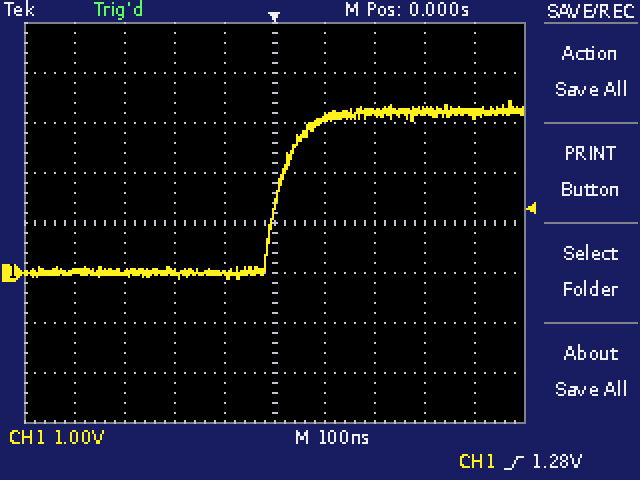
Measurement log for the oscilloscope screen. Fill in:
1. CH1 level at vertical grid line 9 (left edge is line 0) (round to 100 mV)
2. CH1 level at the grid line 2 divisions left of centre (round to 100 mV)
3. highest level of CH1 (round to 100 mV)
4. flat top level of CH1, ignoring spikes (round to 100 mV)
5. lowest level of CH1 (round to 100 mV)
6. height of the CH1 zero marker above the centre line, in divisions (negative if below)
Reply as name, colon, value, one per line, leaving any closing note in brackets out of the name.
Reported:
CH1 level at vertical grid line 9 (left edge is line 0): 3.2 V
CH1 level at the grid line 2 divisions left of centre: 0.0 V
highest level of CH1: 3.4 V
flat top level of CH1, ignoring spikes: 3.2 V
lowest level of CH1: -100 mV
height of the CH1 zero marker above the centre line, in divisions: -1.0 div
